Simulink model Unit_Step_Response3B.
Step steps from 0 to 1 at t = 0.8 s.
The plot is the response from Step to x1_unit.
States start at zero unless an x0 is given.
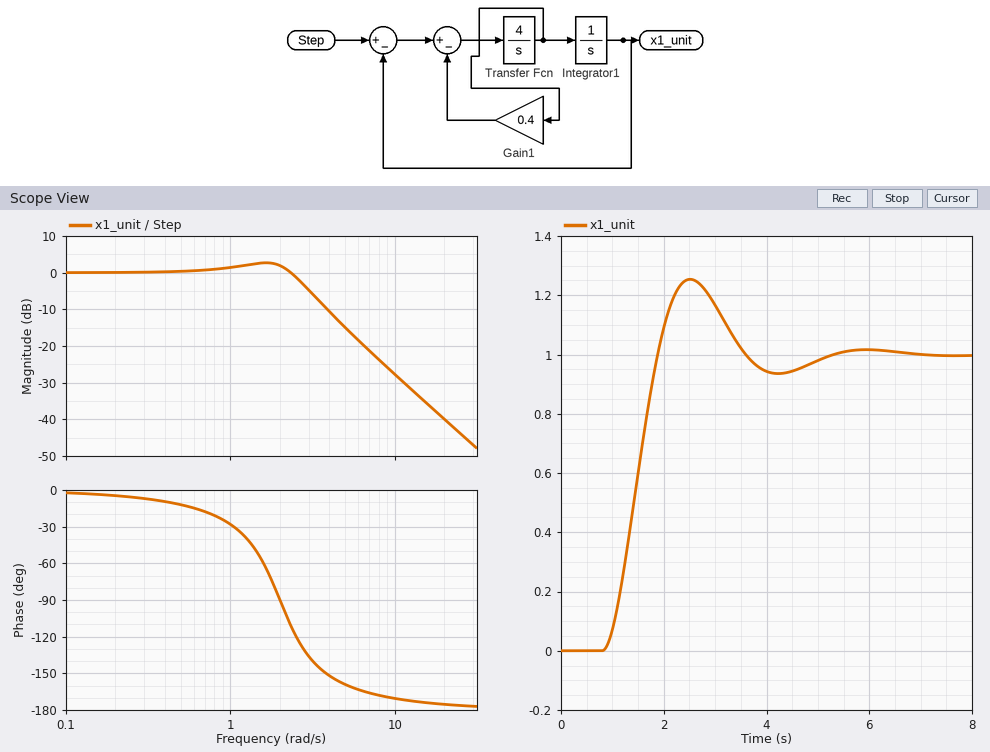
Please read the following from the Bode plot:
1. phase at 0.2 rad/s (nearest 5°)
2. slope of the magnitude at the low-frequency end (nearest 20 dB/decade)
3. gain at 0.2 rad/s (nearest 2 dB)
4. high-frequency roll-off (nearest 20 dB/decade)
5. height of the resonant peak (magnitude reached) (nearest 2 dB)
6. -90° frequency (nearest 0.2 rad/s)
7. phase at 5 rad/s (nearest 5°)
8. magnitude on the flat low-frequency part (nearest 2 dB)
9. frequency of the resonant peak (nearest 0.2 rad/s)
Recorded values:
-5°
0 dB/decade
0 dB
-40 dB/decade
2 dB
2.0 rad/s
-160°
0 dB
1.6 rad/s
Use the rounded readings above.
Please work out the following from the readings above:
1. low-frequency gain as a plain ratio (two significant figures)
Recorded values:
1.0
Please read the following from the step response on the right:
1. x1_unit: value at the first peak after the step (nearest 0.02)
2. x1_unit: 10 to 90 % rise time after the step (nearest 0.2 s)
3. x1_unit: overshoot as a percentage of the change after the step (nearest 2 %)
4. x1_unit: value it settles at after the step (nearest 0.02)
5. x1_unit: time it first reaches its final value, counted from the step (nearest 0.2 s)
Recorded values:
1.26
0.8 s
26 %
1.00
1.0 s
